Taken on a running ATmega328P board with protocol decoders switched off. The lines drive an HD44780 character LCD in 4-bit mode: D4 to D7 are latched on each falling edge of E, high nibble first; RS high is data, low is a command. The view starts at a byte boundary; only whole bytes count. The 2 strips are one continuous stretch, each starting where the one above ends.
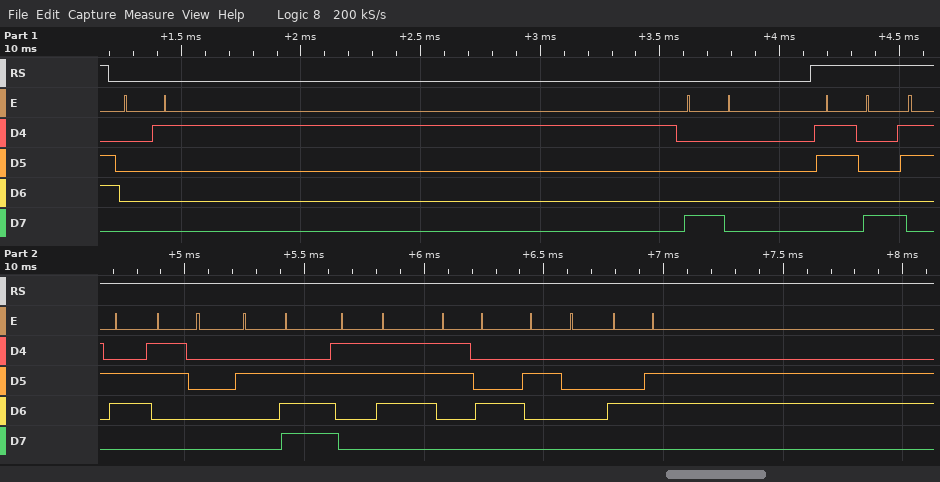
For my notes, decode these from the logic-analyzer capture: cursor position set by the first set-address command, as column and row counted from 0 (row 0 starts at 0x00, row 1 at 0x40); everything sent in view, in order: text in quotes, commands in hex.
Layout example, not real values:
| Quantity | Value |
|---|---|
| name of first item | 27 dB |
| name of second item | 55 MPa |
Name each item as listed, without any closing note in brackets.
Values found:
| Quantity | Value |
|---|---|
| cursor position set by the first set-address command, as column and row counted from 0 | column 0, row 0 |
| everything sent in view, in order: text in quotes, commands in hex | 0x01 0x80 "860.74 F" |
